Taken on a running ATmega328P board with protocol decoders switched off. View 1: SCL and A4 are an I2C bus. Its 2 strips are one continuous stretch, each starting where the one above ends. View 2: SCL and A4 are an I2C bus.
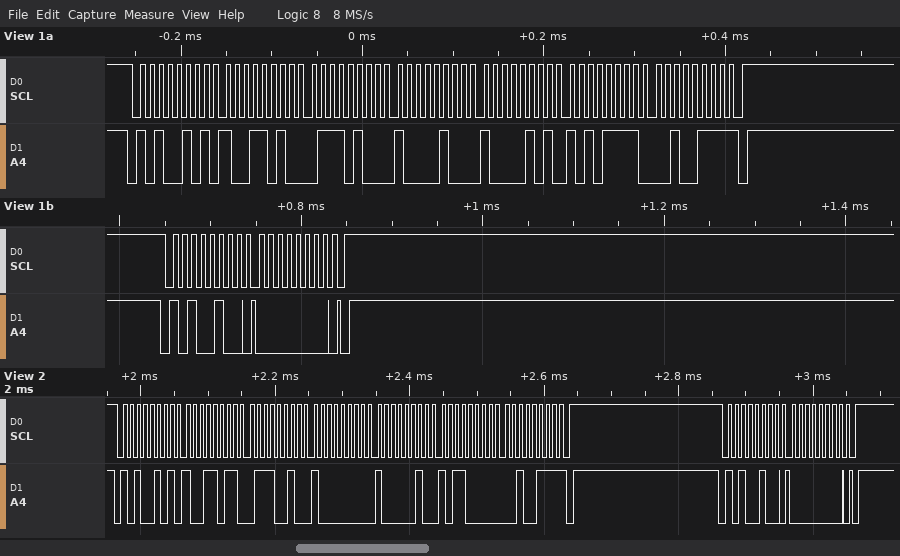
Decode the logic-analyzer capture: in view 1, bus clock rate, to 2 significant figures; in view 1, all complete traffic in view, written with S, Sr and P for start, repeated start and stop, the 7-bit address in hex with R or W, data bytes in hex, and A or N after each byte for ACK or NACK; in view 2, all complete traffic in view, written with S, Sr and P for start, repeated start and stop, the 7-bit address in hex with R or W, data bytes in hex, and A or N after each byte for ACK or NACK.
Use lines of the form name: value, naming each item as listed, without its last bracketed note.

in view 1, bus clock rate, to 2 significant figures: 100 kHz
in view 1, all complete traffic in view, written with S, Sr and P for start, repeated start and stop, the 7-bit address in hex with R or W, data bytes in hex, and A or N after each byte for ACK or NACK: S 52R A 9A A 74 A 84 A 85 A AF A 27 N P S 52W A 00 A P
in view 2, all complete traffic in view, written with S, Sr and P for start, repeated start and stop, the 7-bit address in hex with R or W, data bytes in hex, and A or N after each byte for ACK or NACK: S 52R A 9B A 72 A 80 A 82 A B0 A 27 N P S 52W A 00 A P
